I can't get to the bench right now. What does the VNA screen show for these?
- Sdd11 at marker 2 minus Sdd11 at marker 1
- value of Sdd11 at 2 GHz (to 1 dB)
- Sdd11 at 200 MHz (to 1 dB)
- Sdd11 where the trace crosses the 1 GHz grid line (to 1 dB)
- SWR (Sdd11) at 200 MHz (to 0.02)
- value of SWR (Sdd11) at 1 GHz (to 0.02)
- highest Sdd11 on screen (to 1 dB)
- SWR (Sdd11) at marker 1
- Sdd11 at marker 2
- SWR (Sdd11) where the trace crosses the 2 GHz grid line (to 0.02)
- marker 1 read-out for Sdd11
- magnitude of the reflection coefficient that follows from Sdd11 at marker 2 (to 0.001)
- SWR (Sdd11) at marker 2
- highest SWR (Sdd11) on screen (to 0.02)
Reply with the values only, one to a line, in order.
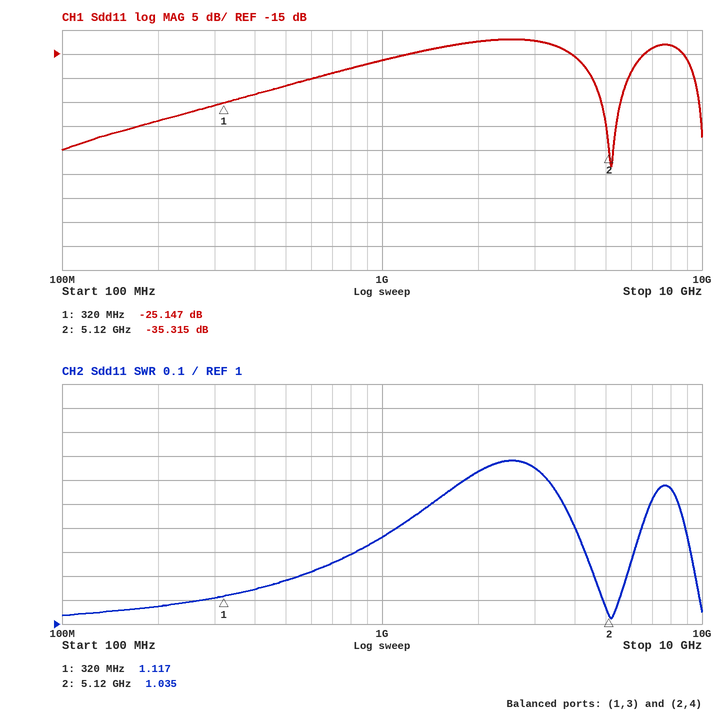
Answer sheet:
-10.168 dB
-12 dB
-29 dB
-16 dB
1.08
1.36
-12 dB
1.117
-35.315 dB
1.64
-25.147 dB
0.017
1.035
1.68
